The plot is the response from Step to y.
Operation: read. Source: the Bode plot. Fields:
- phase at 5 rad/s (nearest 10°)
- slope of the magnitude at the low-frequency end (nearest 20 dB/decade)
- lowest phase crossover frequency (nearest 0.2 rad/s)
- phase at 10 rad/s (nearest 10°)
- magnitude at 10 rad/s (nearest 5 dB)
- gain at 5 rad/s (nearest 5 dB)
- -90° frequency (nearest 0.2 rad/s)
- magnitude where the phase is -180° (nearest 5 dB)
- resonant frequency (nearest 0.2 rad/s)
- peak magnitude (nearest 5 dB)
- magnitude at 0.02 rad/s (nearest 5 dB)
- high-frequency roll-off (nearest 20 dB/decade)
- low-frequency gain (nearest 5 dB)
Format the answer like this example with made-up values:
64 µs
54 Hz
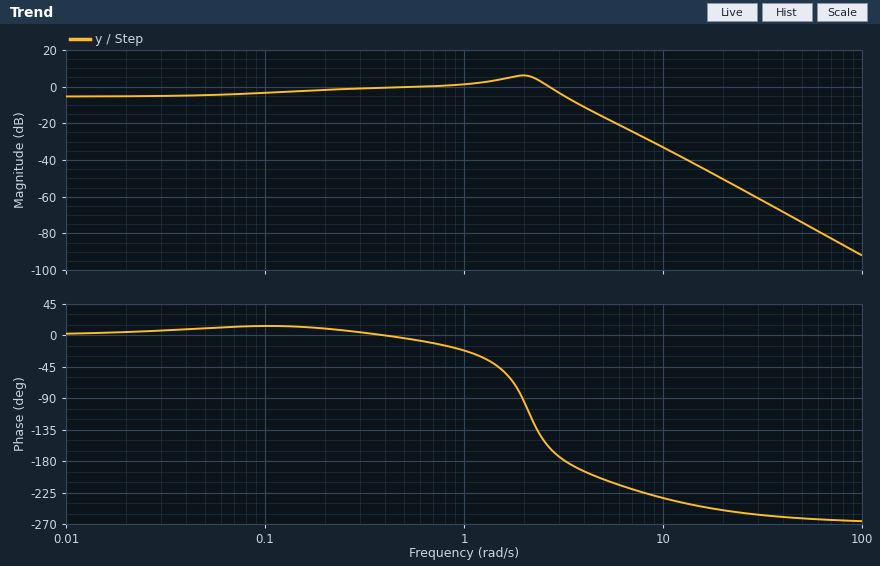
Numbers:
-210°
0 dB/decade
3.2 rad/s
-230°
-35 dB
-15 dB
2.0 rad/s
-5 dB
2.0 rad/s
5 dB
-5 dB
-60 dB/decade
-5 dB
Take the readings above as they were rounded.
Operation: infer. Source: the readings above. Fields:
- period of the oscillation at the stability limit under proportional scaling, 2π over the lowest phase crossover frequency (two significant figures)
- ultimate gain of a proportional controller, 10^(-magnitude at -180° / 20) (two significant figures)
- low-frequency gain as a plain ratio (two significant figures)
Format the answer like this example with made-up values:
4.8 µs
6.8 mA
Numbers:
2.0 s
1.8
0.56
